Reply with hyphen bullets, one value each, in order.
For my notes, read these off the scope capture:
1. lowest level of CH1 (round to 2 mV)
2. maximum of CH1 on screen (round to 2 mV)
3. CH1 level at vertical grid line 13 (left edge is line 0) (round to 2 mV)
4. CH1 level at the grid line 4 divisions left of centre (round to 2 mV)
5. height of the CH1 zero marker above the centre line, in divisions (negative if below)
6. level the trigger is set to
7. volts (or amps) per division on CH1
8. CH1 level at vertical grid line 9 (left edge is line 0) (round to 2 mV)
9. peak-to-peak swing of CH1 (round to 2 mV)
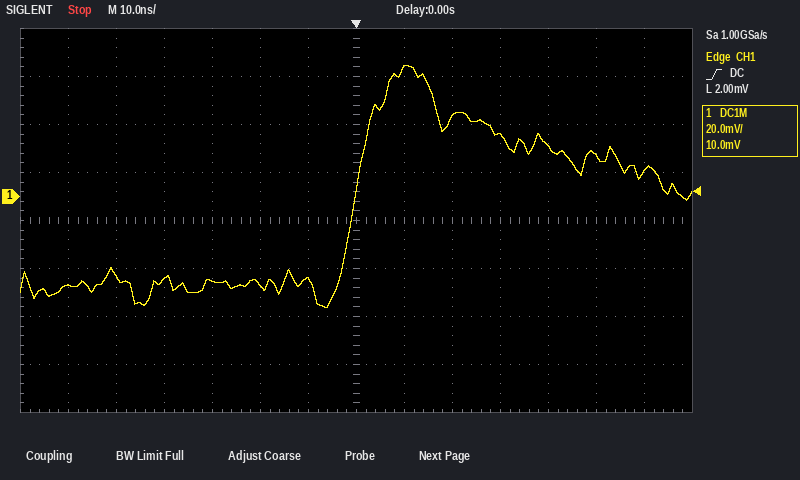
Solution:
- -46 mV
- 54 mV
- 10 mV
- -34 mV
- +0.5 div
- 2.00 mV
- 20 mV
- 34 mV
- 100 mV
